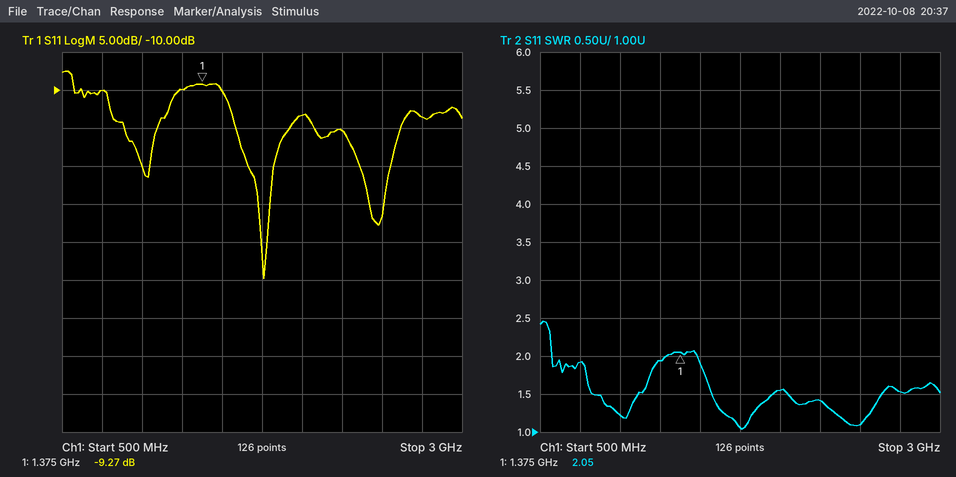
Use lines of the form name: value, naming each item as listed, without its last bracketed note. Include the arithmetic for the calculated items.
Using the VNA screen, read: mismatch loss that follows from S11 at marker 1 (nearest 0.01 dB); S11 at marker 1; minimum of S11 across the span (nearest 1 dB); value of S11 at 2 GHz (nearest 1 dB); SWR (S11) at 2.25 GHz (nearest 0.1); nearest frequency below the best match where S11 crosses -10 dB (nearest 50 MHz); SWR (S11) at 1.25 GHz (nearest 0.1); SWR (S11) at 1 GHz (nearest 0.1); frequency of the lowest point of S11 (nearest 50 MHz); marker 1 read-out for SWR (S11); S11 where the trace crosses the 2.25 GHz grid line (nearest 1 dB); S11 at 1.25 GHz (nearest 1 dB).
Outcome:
mismatch loss that follows from S11 at marker 1: −10 log10(1 − 10^(-9.27/10)) ≈ 0.55 dB
S11 at marker 1: -9.27 dB
minimum of S11 across the span: -35 dB
value of S11 at 2 GHz: -13 dB
SWR (S11) at 2.25 GHz: 1.4
nearest frequency below the best match where S11 crosses -10 dB: 1.50 GHz
SWR (S11) at 1.25 GHz: 1.9
SWR (S11) at 1 GHz: 1.2
frequency of the lowest point of S11: 1.75 GHz
marker 1 read-out for SWR: 2.05
S11 where the trace crosses the 2.25 GHz grid line: -15 dB
S11 at 1.25 GHz: -10 dB
